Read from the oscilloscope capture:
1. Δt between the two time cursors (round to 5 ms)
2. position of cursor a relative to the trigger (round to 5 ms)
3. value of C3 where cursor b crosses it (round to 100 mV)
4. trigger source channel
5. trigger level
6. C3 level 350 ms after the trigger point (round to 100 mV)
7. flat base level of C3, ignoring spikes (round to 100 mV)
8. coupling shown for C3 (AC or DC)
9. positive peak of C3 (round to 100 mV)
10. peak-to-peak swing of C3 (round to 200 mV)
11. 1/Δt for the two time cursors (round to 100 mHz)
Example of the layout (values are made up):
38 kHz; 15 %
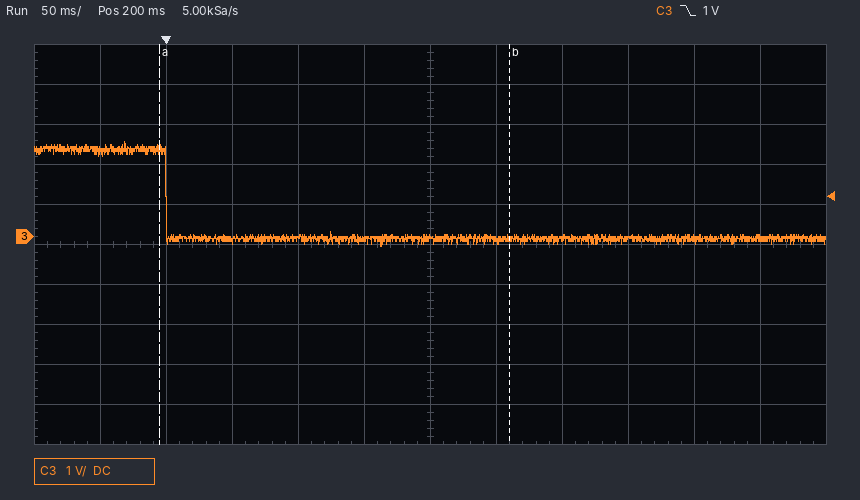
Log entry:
265 ms; -5 ms; 0.0 V; C3; 1 V; -100 mV; -100 mV; DC; 2.4 V; 2.6 V; 3.8 Hz
